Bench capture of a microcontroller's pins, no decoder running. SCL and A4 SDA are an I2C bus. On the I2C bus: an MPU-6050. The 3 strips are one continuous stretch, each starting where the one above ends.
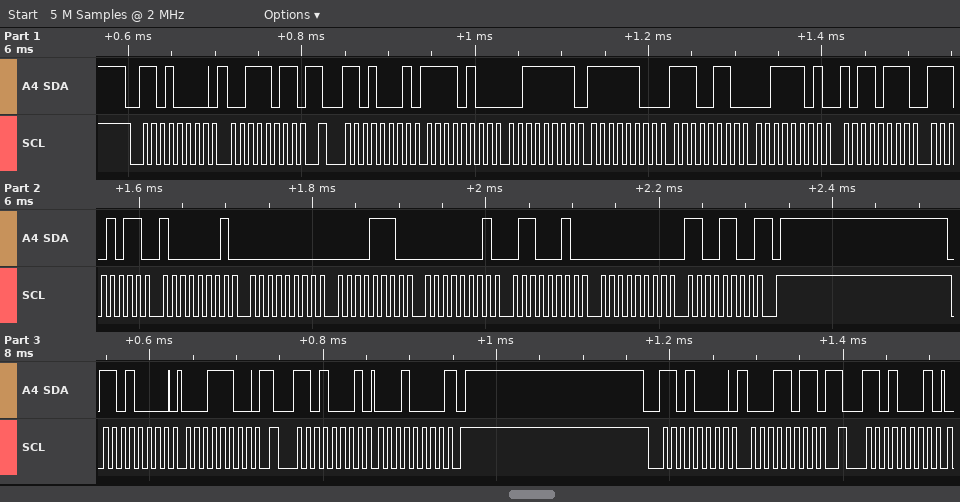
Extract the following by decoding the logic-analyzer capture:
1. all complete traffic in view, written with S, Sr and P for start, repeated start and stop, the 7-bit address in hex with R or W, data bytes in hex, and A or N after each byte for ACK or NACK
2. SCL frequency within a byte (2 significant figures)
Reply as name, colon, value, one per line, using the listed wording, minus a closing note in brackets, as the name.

all complete traffic in view, written with S, Sr and P for start, repeated start and stop, the 7-bit address in hex with R or W, data bytes in hex, and A or N after each byte for ACK or NACK: S 68W A 3B A Sr 68R A F4 A 3F A FC A E6 A 3D A B7 A EB A 81 A 00 A 0E A 01 A 62 A 00 A CC N P S 68W A 1C A Sr 68R A 10 N P S 68W A 1B A Sr 68R A
SCL frequency within a byte: 100 kHz
